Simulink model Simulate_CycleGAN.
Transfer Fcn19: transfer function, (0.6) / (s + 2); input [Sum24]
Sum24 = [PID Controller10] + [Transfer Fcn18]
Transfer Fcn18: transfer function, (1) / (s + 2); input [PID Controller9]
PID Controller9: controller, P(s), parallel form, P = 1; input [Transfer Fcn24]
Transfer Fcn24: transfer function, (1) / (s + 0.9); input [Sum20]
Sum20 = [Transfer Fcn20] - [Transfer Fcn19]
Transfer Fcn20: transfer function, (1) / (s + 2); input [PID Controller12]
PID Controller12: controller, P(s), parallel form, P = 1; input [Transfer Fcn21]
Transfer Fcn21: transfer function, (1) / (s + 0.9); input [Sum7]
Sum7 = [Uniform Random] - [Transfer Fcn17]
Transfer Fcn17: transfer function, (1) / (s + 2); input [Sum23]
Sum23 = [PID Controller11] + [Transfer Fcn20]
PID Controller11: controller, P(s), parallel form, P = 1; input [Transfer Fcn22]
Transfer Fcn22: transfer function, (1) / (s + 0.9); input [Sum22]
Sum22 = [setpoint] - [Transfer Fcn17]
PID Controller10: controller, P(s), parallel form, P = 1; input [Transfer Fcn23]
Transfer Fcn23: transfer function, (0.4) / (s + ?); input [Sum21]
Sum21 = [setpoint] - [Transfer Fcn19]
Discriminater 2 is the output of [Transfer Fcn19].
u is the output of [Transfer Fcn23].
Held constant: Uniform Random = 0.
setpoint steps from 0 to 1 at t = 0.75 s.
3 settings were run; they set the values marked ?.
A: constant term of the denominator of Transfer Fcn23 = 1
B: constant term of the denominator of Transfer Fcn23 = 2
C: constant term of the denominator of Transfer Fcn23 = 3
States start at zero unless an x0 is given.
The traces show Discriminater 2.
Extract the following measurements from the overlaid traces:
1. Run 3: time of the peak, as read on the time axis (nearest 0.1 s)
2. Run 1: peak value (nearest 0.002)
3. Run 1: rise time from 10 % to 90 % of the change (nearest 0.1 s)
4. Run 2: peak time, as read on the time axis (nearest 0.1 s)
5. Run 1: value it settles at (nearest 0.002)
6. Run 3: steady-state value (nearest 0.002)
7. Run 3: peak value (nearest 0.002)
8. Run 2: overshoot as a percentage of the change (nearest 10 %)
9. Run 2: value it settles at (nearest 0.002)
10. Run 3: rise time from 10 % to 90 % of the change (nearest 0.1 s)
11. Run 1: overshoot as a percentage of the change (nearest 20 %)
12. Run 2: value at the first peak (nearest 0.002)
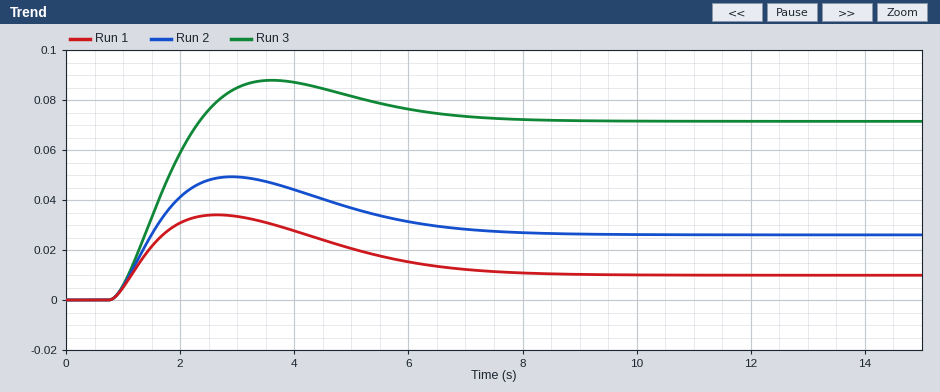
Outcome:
3.6 s
0.034
0.3 s
2.9 s
0.010
0.072
0.088
90 %
0.026
1.1 s
240 %
0.050
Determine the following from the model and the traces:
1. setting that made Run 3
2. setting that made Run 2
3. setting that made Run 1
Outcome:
A
B
C
